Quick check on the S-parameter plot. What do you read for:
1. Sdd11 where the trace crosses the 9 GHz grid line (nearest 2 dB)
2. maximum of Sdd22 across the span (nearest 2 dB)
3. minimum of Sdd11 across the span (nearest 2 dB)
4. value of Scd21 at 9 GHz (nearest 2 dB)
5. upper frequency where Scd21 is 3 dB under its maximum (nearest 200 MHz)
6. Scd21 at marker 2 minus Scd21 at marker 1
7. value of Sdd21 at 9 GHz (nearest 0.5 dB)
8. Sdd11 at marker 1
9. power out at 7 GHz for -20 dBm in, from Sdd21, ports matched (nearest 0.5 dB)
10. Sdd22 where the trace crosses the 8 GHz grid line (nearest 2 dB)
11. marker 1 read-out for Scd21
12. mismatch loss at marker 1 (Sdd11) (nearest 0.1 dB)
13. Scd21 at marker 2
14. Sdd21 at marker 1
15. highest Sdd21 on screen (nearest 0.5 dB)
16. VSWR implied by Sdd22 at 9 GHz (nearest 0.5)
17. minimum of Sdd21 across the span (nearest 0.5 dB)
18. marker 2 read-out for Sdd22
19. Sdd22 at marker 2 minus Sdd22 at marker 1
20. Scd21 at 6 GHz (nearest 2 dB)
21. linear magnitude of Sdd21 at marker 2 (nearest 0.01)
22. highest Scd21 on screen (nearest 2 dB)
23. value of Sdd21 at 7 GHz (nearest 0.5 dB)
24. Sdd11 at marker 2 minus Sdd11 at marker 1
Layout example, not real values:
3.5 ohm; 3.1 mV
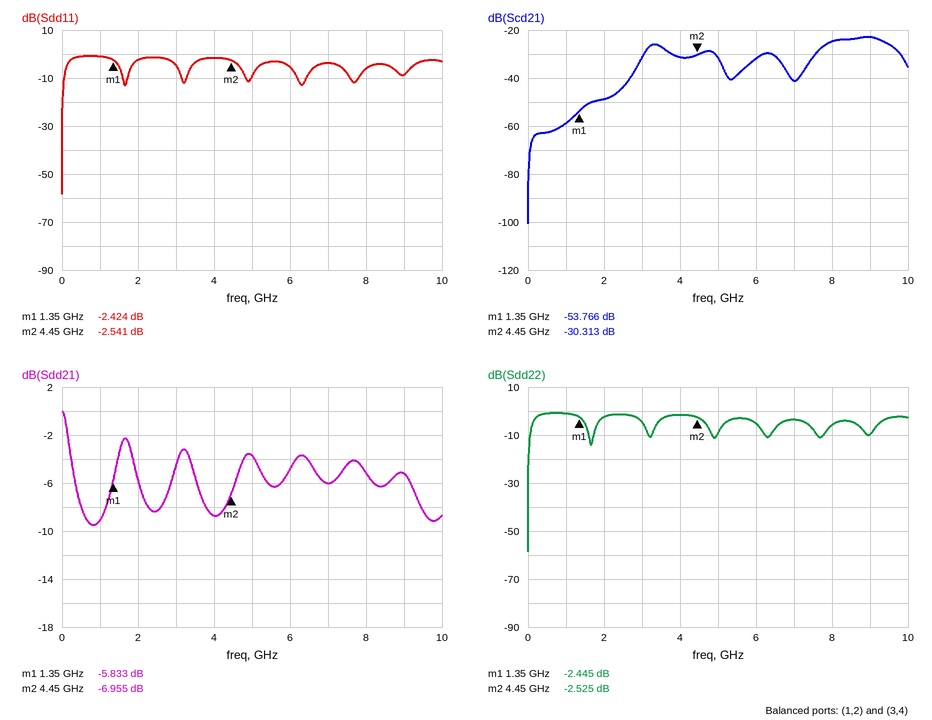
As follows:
-8 dB; 0 dB; -58 dB; -22 dB; 9.4 GHz; 23.453 dB; -5.0 dB; -2.424 dB; -26.0 dBm; -6 dB; -53.766 dB; 3.7 dB; -30.313 dB; -5.833 dB; 0.0 dB; 2.0; -9.5 dB; -2.525 dB; -0.080 dB; -32 dB; 0.45; -22 dB; -6.0 dB; -0.117 dB
